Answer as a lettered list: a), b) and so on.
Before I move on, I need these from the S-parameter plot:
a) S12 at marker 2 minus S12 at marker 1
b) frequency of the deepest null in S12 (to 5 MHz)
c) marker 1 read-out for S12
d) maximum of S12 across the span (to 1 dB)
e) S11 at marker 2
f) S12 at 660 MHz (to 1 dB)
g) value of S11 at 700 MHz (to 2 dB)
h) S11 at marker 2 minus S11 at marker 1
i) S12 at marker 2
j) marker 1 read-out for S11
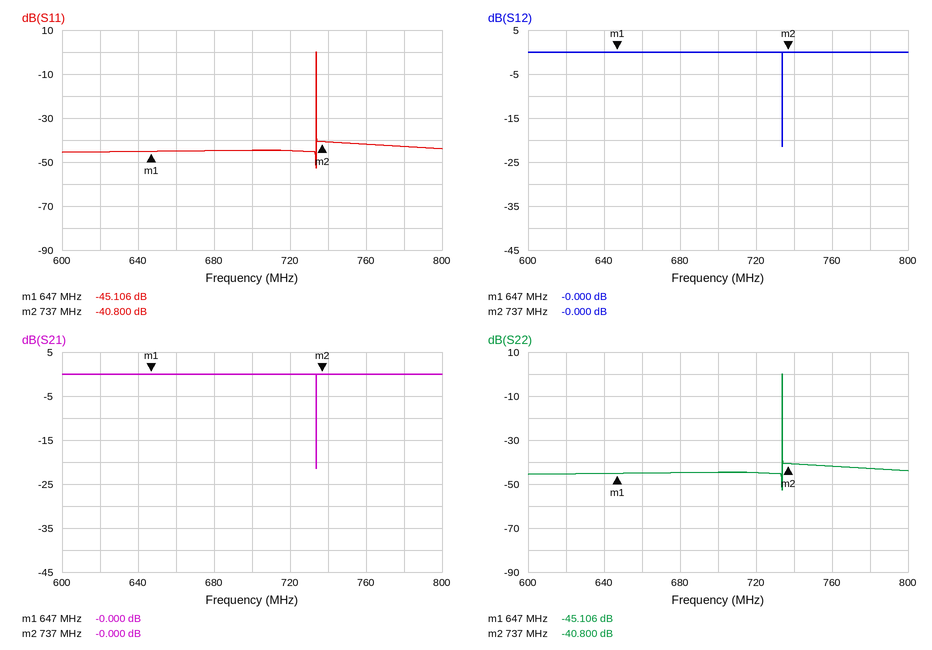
a) 0.000 dB
b) 735 MHz
c) -0.000 dB
d) 0 dB
e) -40.800 dB
f) 0 dB
g) -44 dB
h) 4.306 dB
i) -0.000 dB
j) -45.106 dB
